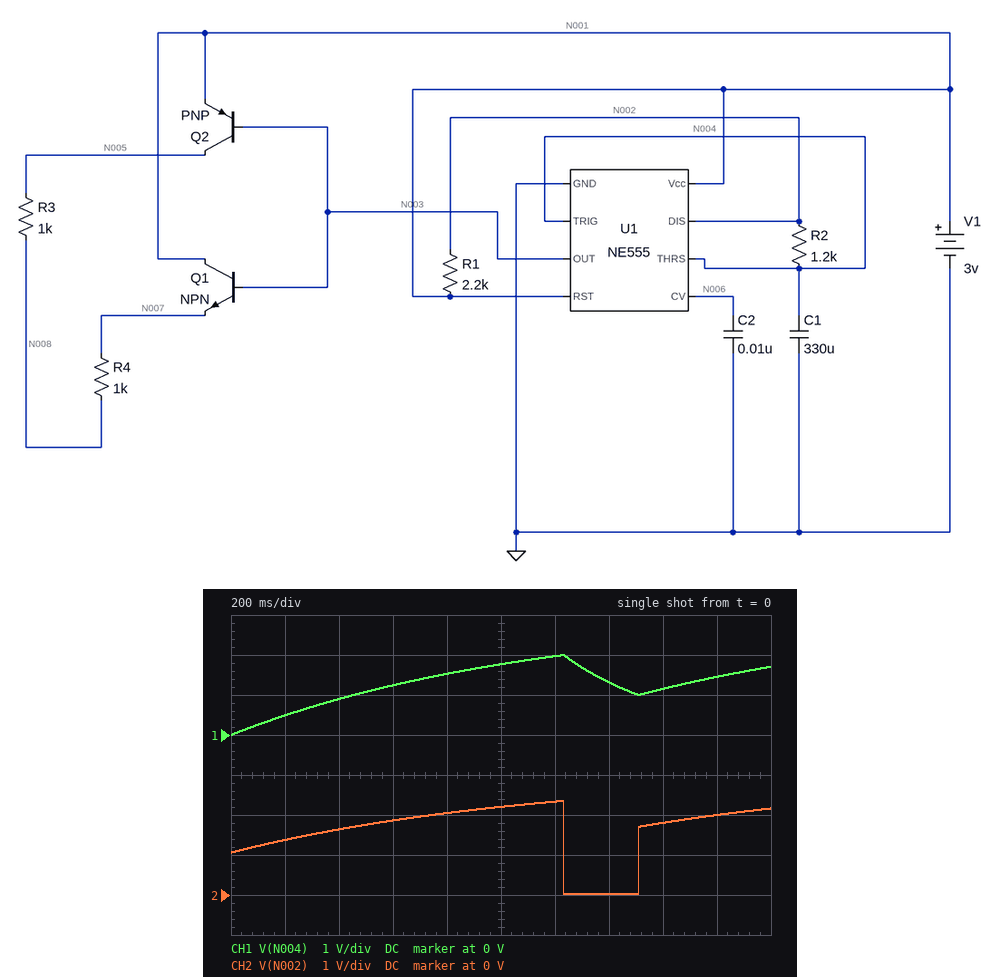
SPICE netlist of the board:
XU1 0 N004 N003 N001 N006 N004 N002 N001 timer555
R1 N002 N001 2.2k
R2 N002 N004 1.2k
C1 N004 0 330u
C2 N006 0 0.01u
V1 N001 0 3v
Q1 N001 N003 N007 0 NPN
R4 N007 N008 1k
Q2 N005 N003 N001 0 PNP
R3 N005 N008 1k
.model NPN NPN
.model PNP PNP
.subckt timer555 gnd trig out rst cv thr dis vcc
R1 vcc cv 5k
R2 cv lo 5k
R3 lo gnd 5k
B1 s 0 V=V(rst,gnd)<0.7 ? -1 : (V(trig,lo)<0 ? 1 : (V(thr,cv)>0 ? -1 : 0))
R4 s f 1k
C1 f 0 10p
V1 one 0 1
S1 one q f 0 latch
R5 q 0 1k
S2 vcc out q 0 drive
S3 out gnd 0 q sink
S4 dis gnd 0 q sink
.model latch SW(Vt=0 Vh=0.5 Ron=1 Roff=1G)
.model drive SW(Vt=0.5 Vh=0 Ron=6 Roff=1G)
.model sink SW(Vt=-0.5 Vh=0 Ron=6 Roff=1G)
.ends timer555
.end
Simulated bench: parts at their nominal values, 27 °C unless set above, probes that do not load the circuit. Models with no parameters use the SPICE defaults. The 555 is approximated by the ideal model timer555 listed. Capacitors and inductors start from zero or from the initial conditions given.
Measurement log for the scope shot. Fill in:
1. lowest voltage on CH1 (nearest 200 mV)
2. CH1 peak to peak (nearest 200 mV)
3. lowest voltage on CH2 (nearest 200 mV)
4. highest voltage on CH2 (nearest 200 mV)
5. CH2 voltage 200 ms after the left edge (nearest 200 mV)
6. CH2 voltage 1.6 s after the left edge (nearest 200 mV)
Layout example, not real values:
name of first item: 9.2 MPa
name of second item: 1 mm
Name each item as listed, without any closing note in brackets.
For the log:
lowest voltage on CH1: 0 V
CH1 peak to peak: 2.0 V
lowest voltage on CH2: 0 V
highest voltage on CH2: 2.4 V
CH2 voltage 200 ms after the left edge: 1.4 V
CH2 voltage 1.6 s after the left edge: 1.8 V
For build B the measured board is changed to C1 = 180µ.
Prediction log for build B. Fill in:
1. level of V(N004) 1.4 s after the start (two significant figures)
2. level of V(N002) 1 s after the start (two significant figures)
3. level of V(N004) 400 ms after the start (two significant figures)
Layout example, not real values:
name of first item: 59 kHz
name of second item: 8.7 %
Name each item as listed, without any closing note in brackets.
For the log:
level of V(N004) 1.4 s after the start: 1.0 V
level of V(N002) 1 s after the start: 2.0 V
level of V(N004) 400 ms after the start: 1.4 V
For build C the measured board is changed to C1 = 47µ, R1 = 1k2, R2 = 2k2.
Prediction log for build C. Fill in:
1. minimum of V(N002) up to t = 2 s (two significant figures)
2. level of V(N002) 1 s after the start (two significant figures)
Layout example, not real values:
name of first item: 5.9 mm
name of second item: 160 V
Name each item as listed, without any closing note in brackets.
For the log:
minimum of V(N002) up to t = 2 s: 18 mV
level of V(N002) 1 s after the start: 2.4 V
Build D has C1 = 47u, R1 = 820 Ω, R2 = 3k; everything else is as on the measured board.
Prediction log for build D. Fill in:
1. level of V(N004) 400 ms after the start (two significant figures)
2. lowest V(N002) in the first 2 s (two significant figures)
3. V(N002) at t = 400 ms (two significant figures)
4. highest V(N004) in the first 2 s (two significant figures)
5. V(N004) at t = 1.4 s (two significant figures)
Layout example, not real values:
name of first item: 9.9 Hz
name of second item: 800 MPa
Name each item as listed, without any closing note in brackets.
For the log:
level of V(N004) 400 ms after the start: 1.9 V
lowest V(N002) in the first 2 s: 24 mV
V(N002) at t = 400 ms: 2.8 V
highest V(N004) in the first 2 s: 2.0 V
V(N004) at t = 1.4 s: 1.1 V
